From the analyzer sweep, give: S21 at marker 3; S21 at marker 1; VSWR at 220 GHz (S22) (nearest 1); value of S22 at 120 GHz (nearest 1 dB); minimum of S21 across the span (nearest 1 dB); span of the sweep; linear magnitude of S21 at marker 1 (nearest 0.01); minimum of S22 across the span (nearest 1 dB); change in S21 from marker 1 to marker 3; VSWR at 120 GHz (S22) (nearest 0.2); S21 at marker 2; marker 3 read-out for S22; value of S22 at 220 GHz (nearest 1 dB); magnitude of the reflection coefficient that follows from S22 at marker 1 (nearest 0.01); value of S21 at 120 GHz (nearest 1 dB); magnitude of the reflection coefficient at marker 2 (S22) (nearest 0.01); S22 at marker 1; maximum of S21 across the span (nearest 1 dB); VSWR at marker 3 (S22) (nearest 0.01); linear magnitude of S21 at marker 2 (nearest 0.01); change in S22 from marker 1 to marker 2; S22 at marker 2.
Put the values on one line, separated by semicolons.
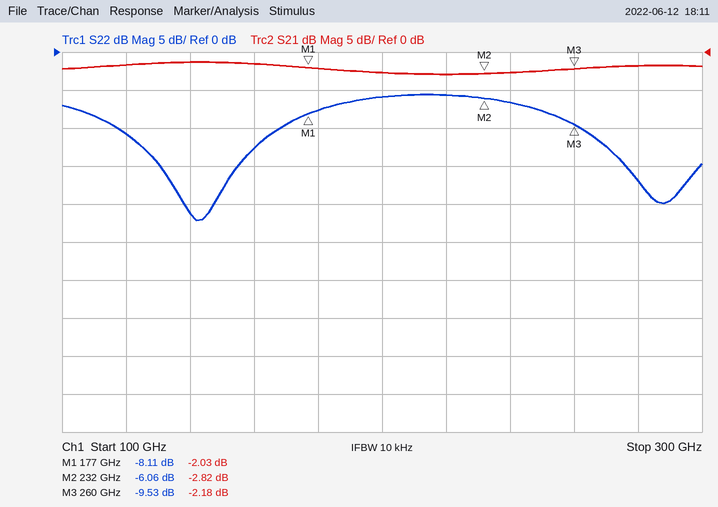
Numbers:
-2.18 dB; -2.03 dB; 3; -11 dB; -3 dB; 200 GHz; 0.79; -22 dB; -0.15 dB; 1.8; -2.82 dB; -9.53 dB; -6 dB; 0.39; -2 dB; 0.50; -8.11 dB; -1 dB; 2.00; 0.72; 2.05 dB; -6.06 dB
